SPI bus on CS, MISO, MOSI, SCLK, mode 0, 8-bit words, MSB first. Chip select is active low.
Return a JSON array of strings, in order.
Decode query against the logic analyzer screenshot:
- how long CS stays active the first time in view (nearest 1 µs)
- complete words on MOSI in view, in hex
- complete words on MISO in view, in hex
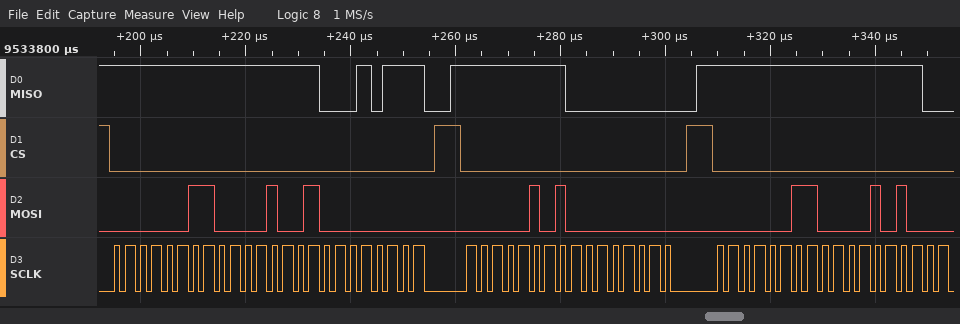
["62 µs", "03, 09, 00, 05, 00, 03, 0A", "FF, FF, 17, FF, 00, FF, FF"]
